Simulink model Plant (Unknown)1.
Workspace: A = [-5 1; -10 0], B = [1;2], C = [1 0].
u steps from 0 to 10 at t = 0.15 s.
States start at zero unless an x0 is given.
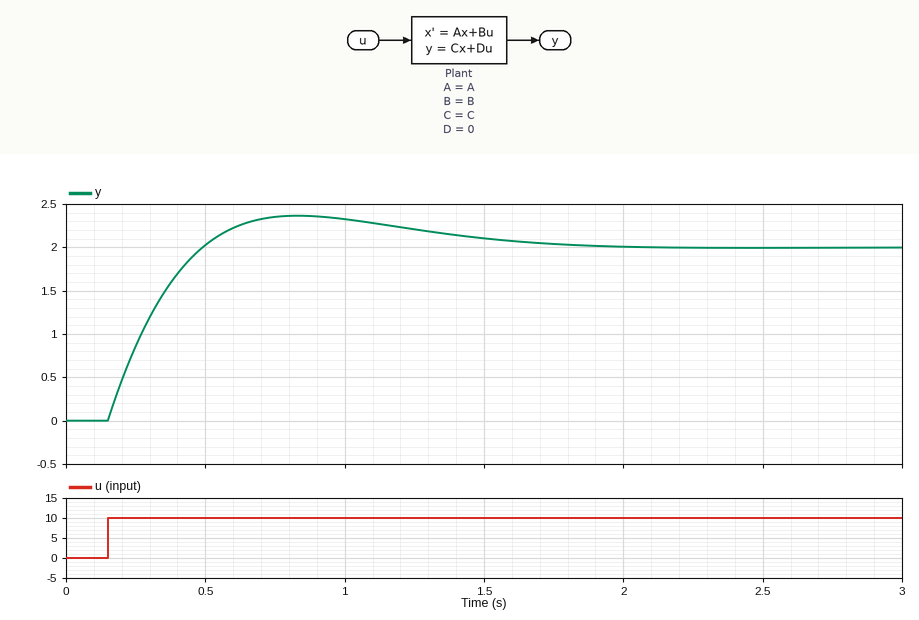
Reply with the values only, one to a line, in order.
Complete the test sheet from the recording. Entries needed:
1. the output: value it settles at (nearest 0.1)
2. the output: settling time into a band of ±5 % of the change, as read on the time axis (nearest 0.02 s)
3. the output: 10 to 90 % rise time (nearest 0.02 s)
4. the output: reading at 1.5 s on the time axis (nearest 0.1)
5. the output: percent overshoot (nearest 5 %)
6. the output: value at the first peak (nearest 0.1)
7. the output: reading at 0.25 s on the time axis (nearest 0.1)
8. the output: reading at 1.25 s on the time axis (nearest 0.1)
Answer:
2.0
1.52 s
0.26 s
2.1
20 %
2.4
0.9
2.2
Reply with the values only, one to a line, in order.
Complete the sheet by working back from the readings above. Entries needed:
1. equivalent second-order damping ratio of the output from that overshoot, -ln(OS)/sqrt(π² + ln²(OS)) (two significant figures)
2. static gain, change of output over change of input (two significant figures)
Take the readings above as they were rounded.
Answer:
0.46
0.20
